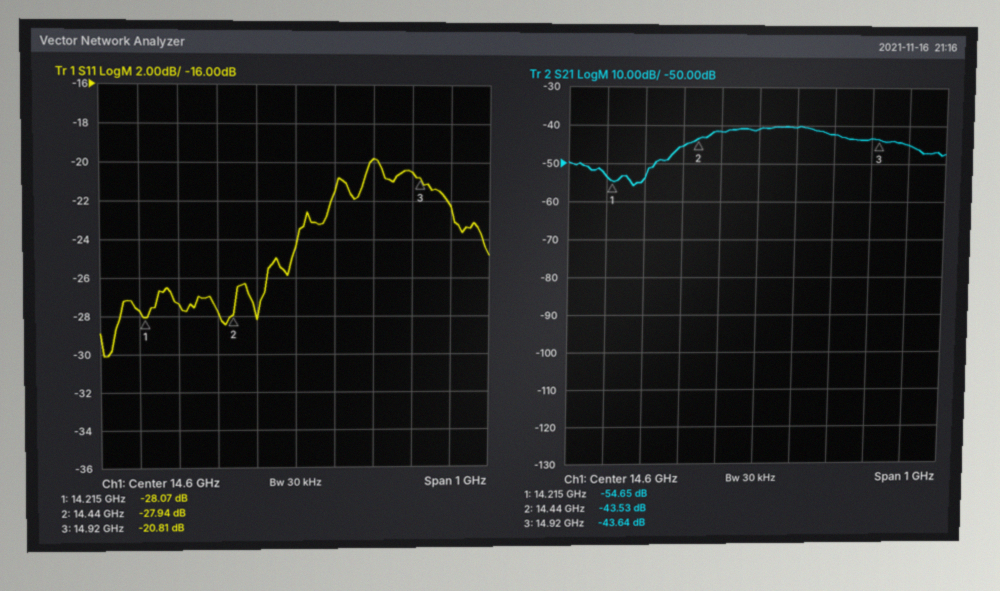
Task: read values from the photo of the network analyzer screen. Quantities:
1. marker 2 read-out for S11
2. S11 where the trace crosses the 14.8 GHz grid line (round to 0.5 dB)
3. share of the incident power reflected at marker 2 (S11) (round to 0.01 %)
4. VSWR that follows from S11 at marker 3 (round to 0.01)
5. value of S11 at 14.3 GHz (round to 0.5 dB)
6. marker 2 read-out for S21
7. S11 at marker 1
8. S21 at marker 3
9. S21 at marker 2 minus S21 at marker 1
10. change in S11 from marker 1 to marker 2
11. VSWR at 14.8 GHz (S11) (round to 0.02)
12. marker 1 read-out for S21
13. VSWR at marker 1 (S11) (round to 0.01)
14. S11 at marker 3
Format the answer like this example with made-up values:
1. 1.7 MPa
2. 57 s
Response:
1. -27.94 dB
2. -20.0 dB
3. 0.16 %
4. 1.20
5. -27.5 dB
6. -43.53 dB
7. -28.07 dB
8. -43.64 dB
9. 11.12 dB
10. 0.13 dB
11. 1.22
12. -54.65 dB
13. 1.08
14. -20.81 dB
